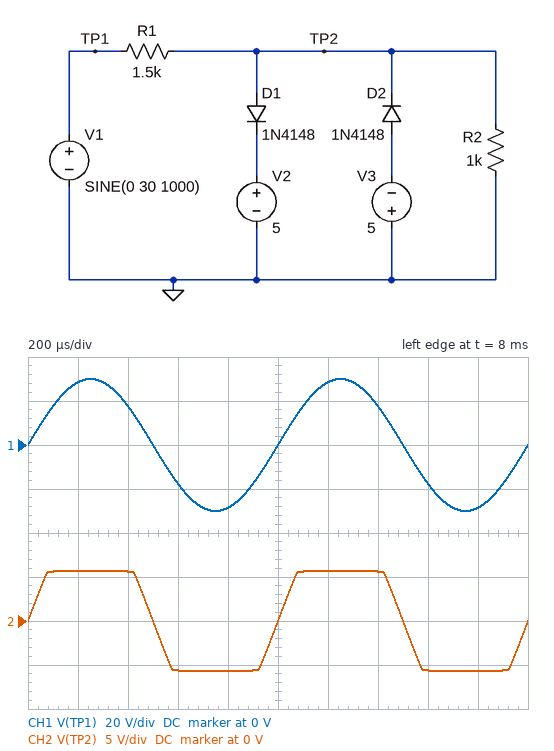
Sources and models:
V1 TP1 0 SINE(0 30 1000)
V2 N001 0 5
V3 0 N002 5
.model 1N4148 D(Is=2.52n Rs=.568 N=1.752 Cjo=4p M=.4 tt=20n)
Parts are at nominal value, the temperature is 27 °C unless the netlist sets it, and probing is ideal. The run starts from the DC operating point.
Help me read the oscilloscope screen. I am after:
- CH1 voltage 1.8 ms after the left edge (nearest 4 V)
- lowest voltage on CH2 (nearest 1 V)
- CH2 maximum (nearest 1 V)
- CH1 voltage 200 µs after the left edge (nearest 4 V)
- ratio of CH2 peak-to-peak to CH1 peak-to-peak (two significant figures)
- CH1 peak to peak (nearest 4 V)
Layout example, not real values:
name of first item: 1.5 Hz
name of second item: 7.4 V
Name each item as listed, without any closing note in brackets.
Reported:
CH1 voltage 1.8 ms after the left edge: -28 V
lowest voltage on CH2: -6 V
CH2 maximum: 6 V
CH1 voltage 200 µs after the left edge: 28 V
ratio of CH2 peak-to-peak to CH1 peak-to-peak: 0.19
CH1 peak to peak: 60 V
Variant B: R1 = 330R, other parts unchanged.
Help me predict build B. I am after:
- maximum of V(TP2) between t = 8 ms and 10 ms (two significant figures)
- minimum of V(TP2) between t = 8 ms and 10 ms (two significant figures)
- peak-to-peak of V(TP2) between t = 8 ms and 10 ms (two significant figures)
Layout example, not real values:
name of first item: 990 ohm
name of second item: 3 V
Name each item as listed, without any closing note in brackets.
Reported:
maximum of V(TP2) between t = 8 ms and 10 ms: 5.8 V
minimum of V(TP2) between t = 8 ms and 10 ms: -5.8 V
peak-to-peak of V(TP2) between t = 8 ms and 10 ms: 12 V
